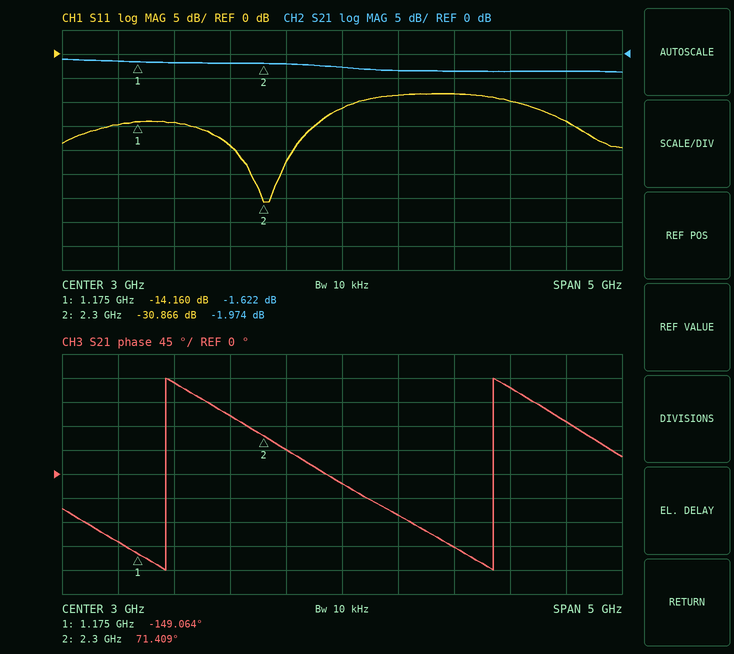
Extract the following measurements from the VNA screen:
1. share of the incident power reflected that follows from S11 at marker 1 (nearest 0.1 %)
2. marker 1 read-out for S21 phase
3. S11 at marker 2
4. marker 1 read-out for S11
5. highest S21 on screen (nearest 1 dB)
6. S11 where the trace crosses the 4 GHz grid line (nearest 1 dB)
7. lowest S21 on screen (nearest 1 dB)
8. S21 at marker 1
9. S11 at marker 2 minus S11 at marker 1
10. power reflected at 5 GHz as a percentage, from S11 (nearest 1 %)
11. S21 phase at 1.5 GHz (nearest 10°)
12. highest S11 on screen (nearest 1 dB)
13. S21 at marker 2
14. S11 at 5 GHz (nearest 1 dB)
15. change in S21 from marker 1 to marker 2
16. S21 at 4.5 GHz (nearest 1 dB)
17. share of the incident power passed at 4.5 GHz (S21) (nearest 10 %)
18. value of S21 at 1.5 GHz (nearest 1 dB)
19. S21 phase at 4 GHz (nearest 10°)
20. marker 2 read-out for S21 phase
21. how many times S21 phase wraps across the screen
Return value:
3.8 %
-149.064°
-30.866 dB
-14.160 dB
-1 dB
-8 dB
-4 dB
-1.622 dB
-16.706 dB
4 %
170°
-8 dB
-1.974 dB
-14 dB
-0.352 dB
-4 dB
40 %
-2 dB
-140°
71.409°
2
